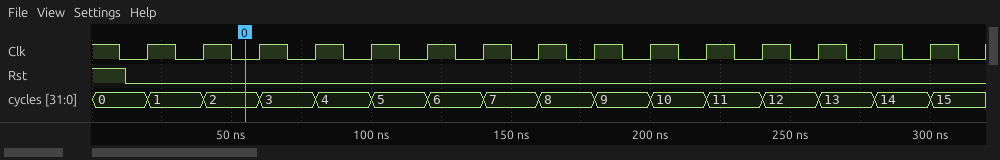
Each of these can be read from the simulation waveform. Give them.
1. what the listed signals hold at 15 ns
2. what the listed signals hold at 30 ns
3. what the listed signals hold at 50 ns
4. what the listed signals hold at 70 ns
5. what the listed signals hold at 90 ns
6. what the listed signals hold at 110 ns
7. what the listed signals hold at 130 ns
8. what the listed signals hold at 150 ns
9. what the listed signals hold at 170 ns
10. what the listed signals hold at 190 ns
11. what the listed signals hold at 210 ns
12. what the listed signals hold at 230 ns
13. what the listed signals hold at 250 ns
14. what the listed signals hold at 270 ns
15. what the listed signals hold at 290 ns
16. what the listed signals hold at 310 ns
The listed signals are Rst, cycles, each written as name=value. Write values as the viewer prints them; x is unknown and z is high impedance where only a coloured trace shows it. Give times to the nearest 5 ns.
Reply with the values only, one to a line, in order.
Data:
Rst=0, cycles=0
Rst=0, cycles=1
Rst=0, cycles=2
Rst=0, cycles=3
Rst=0, cycles=4
Rst=0, cycles=5
Rst=0, cycles=6
Rst=0, cycles=7
Rst=0, cycles=8
Rst=0, cycles=9
Rst=0, cycles=10
Rst=0, cycles=11
Rst=0, cycles=12
Rst=0, cycles=13
Rst=0, cycles=14
Rst=0, cycles=15
